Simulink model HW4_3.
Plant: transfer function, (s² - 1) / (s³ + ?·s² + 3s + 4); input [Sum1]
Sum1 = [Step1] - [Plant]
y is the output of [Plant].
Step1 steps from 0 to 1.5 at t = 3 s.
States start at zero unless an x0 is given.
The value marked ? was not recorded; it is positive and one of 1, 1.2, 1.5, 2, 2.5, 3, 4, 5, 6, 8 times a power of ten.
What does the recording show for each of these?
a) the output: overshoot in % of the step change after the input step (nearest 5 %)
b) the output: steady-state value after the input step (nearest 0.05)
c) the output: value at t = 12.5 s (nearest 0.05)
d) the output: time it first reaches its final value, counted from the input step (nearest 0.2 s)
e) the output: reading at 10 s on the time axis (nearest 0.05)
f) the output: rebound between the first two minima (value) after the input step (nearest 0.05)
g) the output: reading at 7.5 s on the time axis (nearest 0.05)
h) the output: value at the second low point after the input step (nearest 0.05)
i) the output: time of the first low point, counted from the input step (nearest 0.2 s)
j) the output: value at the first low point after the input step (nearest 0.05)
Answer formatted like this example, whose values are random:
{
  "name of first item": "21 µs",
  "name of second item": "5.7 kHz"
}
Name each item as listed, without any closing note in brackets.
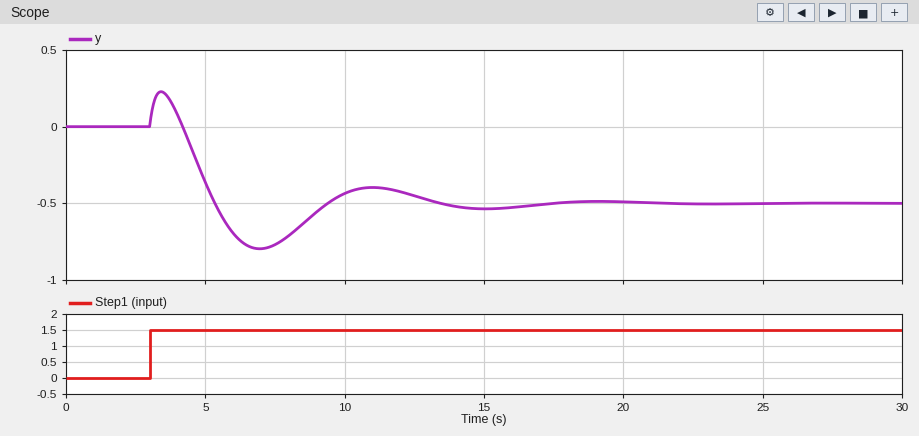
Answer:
{
  "the output: overshoot in % of the step change after the input step": "60 %",
  "the output: steady-state value after the input step": "-0.50",
  "the output: value at t = 12.5 s": "-0.45",
  "the output: time it first reaches its final value, counted from the input step": "2.4 s",
  "the output: reading at 10 s on the time axis": "-0.45",
  "the output: rebound between the first two minima (value) after the input step": "-0.40",
  "the output: reading at 7.5 s on the time axis": "-0.75",
  "the output: value at the second low point after the input step": "-0.55",
  "the output: time of the first low point, counted from the input step": "4.0 s",
  "the output: value at the first low point after the input step": "-0.80"
}
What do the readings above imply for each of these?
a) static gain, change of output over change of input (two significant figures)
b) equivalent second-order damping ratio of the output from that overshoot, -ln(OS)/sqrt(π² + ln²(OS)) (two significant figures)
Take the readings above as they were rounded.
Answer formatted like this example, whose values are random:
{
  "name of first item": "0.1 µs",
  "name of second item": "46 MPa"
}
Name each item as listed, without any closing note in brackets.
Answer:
{
  "static gain, change of output over change of input": "-0.33",
  "equivalent second-order damping ratio of the output from that overshoot, -ln(OS)/sqrt(π² + ln²(OS))": "0.16"
}
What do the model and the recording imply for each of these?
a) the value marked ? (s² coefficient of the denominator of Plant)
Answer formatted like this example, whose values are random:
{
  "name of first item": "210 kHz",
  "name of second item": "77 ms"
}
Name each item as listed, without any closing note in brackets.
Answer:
{
  "the value marked ?": "4"
}
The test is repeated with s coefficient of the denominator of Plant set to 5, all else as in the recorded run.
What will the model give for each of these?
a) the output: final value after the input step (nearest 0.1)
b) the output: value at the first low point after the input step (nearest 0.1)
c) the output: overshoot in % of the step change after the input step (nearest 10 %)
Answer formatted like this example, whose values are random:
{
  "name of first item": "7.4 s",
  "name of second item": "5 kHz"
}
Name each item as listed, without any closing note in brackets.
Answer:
{
  "the output: final value after the input step": "-0.5",
  "the output: value at the first low point after the input step": "-0.6",
  "the output: overshoot in % of the step change after the input step": "20 %"
}
